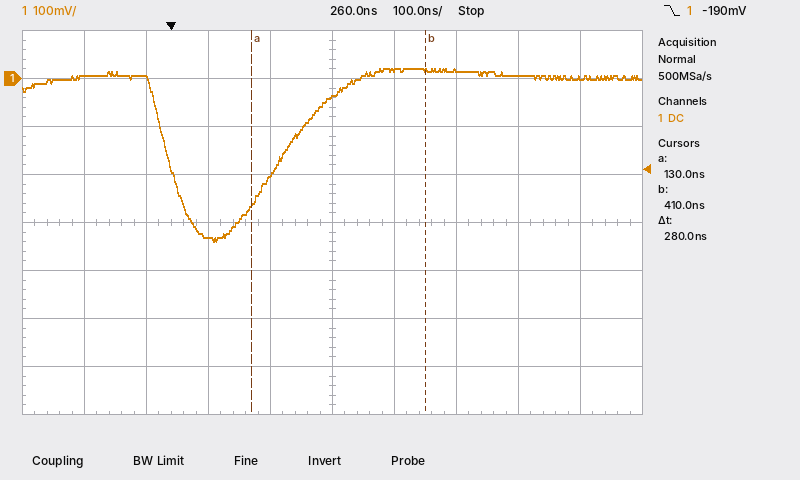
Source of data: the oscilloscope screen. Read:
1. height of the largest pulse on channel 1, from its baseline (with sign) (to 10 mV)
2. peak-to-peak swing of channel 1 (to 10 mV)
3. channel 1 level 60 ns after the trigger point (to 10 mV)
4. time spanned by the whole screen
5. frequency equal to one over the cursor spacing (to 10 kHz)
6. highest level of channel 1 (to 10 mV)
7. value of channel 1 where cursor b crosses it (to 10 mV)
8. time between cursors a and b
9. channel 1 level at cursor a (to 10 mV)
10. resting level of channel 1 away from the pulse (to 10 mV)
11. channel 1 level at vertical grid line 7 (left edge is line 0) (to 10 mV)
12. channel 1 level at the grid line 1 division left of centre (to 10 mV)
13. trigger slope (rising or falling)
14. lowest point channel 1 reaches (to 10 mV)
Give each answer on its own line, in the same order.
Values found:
-340 mV
360 mV
-330 mV
1 µs
3.57 MHz
20 mV
20 mV
280 ns
-270 mV
0 mV
20 mV
-200 mV
falling
-340 mV
